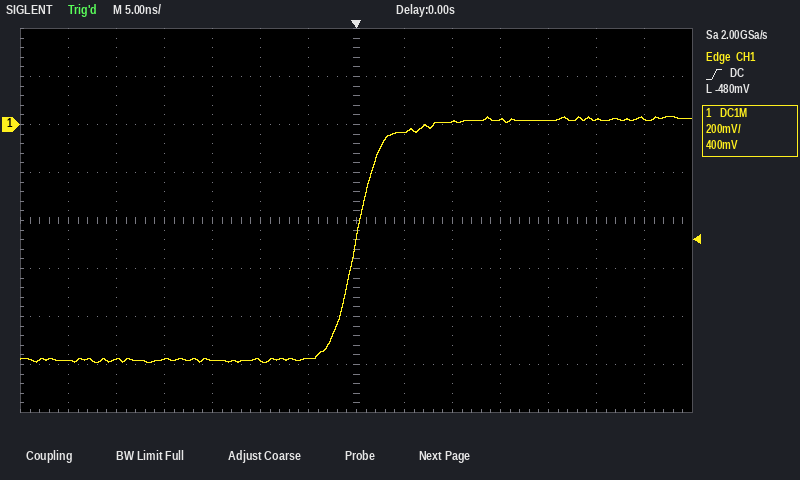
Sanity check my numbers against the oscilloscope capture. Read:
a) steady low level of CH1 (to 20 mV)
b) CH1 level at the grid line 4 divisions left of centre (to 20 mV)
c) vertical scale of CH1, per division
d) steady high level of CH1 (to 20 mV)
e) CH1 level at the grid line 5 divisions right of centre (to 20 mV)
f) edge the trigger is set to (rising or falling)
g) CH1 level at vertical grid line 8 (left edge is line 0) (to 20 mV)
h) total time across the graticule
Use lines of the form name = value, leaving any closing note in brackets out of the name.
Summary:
steady low level of CH1 = -980 mV
CH1 level at the grid line 4 divisions left of centre = -980 mV
vertical scale of CH1, per division = 200 mV
steady high level of CH1 = 20 mV
CH1 level at the grid line 5 divisions right of centre = 20 mV
edge the trigger is set to = rising
CH1 level at vertical grid line 8 (left edge is line 0) = -40 mV
total time across the graticule = 70 ns
